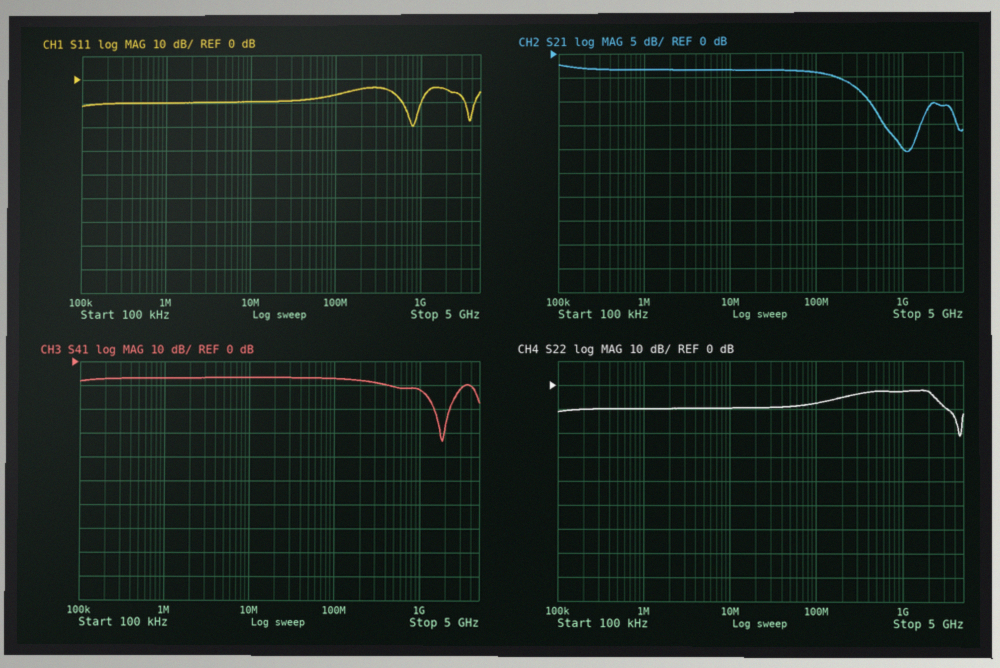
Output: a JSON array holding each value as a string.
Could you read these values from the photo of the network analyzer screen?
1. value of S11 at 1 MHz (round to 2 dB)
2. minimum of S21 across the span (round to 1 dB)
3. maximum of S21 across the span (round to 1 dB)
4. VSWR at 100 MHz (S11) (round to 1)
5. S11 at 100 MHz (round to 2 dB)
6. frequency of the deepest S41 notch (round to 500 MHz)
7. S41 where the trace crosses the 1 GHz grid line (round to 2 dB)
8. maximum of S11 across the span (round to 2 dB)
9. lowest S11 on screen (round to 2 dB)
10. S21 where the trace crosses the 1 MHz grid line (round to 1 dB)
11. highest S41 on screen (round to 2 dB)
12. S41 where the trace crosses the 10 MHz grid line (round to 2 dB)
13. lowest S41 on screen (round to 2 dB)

["-10 dB", "-21 dB", "-2 dB", "3", "-6 dB", "2.0 GHz", "-12 dB", "-4 dB", "-20 dB", "-3 dB", "-6 dB", "-6 dB", "-34 dB"]
